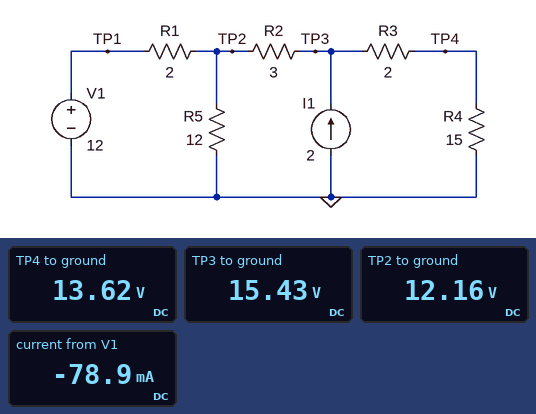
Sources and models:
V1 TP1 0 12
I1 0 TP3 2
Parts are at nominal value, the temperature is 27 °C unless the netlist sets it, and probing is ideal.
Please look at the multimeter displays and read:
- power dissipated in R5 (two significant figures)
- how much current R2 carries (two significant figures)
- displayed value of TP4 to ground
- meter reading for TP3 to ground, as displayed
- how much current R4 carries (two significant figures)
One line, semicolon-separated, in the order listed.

12 W; 1.1 A; 13.62 V; 15.43 V; 910 mA
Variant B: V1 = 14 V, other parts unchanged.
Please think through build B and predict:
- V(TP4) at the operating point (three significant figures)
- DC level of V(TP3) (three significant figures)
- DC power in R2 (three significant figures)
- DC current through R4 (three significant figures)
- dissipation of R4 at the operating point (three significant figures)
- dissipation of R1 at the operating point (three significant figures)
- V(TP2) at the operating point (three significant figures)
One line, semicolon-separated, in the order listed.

14.8 V; 16.8 V; 3.08 W; 987 mA; 14.6 W; 34.6 mW; 13.7 V
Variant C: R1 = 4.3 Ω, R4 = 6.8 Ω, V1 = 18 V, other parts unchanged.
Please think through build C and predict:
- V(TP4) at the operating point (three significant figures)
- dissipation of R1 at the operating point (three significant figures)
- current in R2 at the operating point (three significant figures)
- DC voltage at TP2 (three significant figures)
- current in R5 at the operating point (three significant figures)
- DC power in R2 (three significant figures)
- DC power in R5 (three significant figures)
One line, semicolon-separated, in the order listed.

11.6 V; 3.41 W; 291 mA; 14.2 V; 1.18 A; 253 mW; 16.7 W
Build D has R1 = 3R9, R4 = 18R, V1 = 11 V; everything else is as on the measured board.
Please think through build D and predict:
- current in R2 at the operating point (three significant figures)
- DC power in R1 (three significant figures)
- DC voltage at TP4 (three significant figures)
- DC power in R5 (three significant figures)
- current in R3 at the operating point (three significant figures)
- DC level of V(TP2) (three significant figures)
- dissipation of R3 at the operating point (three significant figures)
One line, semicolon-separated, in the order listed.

1.22 A; 207 mW; 14.0 V; 11.8 W; 778 mA; 11.9 V; 1.21 W
